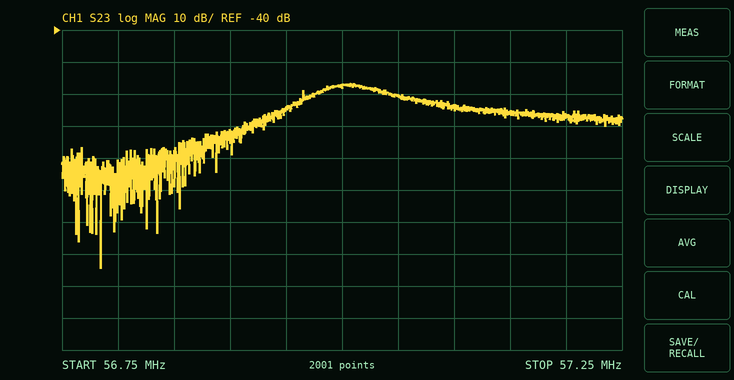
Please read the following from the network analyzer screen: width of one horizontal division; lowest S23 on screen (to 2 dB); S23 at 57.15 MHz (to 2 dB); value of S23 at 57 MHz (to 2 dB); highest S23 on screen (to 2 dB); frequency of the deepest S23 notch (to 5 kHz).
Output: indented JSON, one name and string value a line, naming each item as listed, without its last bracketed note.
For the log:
{
  "width of one horizontal division": "50 kHz",
  "lowest S23 on screen": "-114 dB",
  "S23 at 57.15 MHz": "-66 dB",
  "value of S23 at 57 MHz": "-58 dB",
  "highest S23 on screen": "-56 dB",
  "frequency of the deepest S23 notch": "56.785 MHz"
}
